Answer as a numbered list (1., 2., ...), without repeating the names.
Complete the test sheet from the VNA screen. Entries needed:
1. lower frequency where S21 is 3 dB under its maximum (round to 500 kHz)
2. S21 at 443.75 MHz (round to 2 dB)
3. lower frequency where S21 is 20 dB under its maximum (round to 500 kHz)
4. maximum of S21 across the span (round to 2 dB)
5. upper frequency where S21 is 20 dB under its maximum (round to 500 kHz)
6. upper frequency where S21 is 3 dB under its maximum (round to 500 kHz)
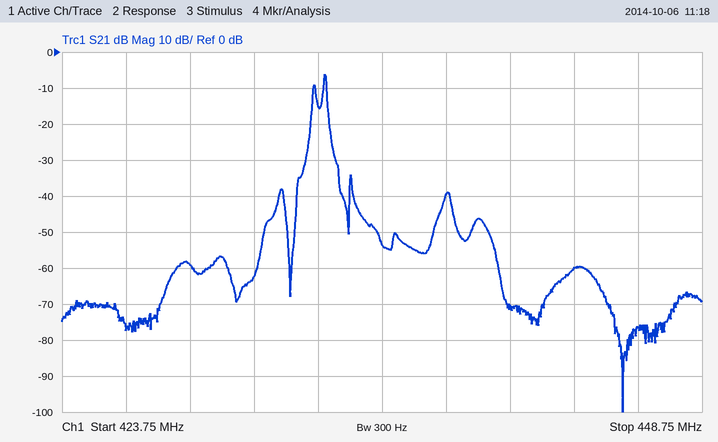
1. 434.0 MHz
2. -60 dB
3. 433.5 MHz
4. -6 dB
5. 434.5 MHz
6. 434.0 MHz
